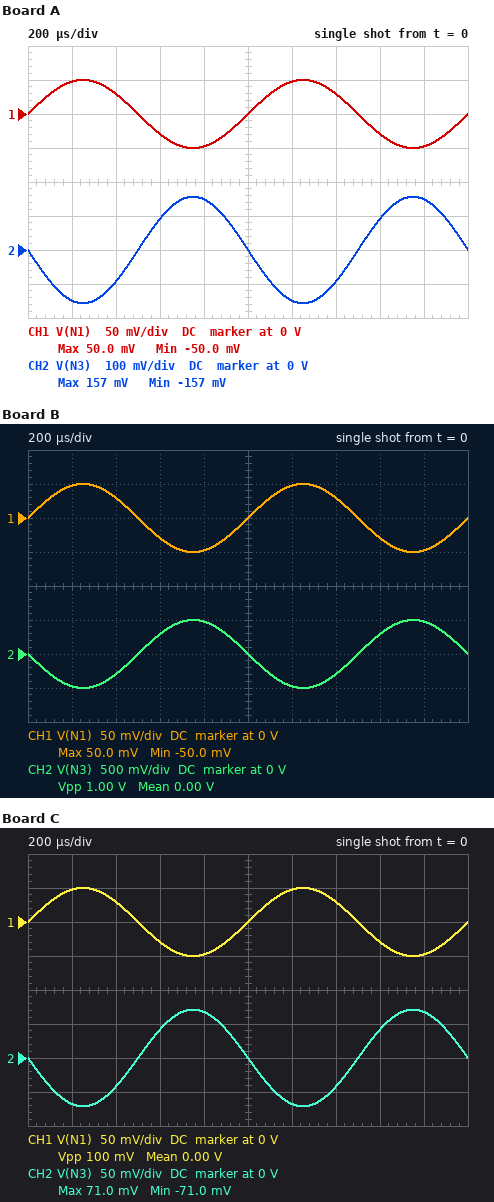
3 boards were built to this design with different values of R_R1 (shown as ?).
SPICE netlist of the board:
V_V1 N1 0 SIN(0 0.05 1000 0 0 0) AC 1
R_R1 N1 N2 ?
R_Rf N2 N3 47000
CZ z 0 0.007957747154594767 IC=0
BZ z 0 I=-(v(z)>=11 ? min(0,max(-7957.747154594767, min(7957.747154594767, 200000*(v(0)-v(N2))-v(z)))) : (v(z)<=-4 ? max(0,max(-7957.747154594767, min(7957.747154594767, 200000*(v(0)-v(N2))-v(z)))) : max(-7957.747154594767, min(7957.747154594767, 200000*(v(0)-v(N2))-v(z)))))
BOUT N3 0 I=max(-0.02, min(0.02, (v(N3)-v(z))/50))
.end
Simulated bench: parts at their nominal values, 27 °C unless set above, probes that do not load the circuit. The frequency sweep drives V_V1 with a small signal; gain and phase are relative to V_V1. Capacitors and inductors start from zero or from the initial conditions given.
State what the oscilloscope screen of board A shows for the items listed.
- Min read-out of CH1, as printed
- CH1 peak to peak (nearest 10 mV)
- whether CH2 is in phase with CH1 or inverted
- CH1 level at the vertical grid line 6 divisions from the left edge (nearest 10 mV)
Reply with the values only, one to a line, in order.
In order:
-50.0 mV
100 mV
inverted
50 mV
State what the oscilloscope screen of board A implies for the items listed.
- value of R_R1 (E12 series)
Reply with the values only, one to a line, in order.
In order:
15 kΩ
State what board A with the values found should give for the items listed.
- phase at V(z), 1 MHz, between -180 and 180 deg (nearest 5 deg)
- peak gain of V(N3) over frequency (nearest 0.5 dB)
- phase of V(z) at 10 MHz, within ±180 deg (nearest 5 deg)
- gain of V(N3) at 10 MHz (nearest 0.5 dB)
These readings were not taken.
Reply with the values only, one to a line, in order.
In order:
135 deg
10.0 dB
95 deg
-10.5 dB
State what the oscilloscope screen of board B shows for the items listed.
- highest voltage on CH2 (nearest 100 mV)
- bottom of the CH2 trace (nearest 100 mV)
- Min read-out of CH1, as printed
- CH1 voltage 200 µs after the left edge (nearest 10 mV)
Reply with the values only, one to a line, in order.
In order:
500 mV
-500 mV
-50.0 mV
50 mV
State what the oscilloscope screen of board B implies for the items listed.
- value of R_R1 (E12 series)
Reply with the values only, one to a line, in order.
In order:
4.7 kΩ
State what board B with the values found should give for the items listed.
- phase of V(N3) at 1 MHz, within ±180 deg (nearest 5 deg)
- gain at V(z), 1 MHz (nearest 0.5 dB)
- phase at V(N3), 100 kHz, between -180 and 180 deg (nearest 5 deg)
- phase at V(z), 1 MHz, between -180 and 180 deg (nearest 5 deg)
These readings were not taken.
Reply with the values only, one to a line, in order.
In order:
110 deg
10.5 dB
165 deg
110 deg
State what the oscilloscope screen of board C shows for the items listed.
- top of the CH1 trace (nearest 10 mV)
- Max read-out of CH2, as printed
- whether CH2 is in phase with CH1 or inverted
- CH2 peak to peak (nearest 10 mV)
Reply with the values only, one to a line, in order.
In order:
50 mV
71.0 mV
inverted
140 mV
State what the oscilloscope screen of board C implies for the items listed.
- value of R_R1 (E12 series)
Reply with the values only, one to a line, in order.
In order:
33 kΩ
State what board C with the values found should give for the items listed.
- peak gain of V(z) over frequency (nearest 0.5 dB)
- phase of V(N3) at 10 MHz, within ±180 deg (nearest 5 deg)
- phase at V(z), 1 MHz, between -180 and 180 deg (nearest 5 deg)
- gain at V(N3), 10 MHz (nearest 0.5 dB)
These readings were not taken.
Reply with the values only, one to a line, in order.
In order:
3.0 dB
100 deg
150 deg
-12.5 dB
